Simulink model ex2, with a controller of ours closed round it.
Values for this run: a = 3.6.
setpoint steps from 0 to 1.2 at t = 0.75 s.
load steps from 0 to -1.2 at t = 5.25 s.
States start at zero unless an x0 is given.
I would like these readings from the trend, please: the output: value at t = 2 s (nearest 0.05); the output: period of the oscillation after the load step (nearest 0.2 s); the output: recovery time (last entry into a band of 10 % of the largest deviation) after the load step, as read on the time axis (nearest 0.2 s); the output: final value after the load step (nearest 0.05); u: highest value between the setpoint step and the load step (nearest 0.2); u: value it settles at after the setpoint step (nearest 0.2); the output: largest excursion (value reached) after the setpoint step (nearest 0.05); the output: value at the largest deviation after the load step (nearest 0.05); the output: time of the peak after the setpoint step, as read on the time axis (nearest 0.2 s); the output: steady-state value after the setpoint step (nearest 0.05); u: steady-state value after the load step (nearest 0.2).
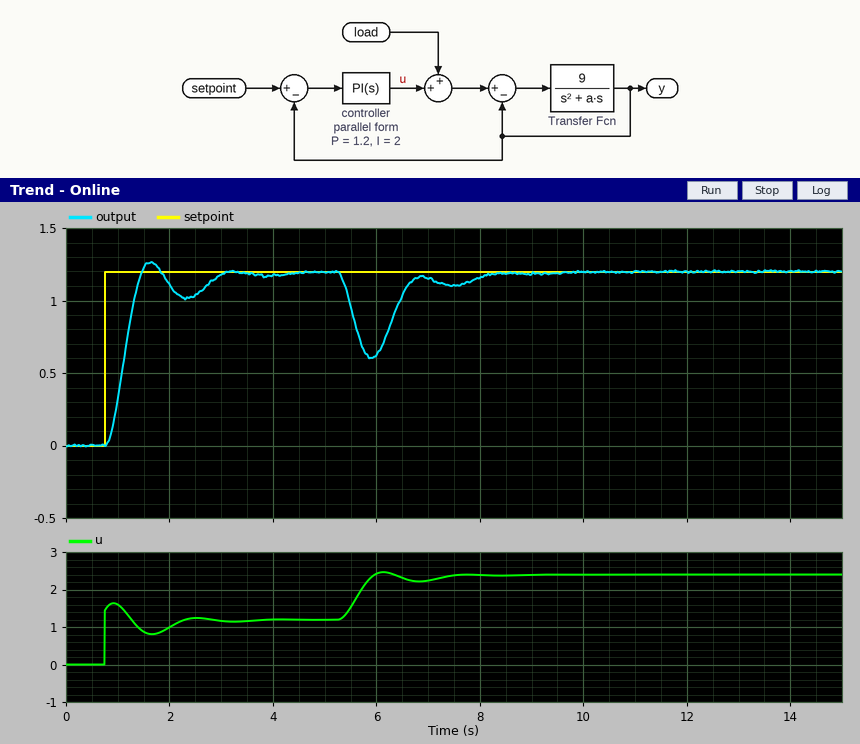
1.10
1.6 s
7.8 s
1.20
1.6
1.2
1.25
0.60
1.6 s
1.20
2.4
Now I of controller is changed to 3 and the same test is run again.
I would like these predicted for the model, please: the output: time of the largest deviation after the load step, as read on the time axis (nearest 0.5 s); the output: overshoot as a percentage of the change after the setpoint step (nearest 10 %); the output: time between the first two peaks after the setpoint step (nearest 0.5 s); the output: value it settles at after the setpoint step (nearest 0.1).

6.0 s
20 %
1.5 s
1.2
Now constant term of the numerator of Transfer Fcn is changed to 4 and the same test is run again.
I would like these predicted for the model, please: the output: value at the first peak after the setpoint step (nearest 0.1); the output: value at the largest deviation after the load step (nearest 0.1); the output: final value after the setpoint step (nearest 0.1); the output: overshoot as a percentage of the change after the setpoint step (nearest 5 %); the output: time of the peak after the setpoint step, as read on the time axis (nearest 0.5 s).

1.4
0.7
1.2
15 %
2.5 s
